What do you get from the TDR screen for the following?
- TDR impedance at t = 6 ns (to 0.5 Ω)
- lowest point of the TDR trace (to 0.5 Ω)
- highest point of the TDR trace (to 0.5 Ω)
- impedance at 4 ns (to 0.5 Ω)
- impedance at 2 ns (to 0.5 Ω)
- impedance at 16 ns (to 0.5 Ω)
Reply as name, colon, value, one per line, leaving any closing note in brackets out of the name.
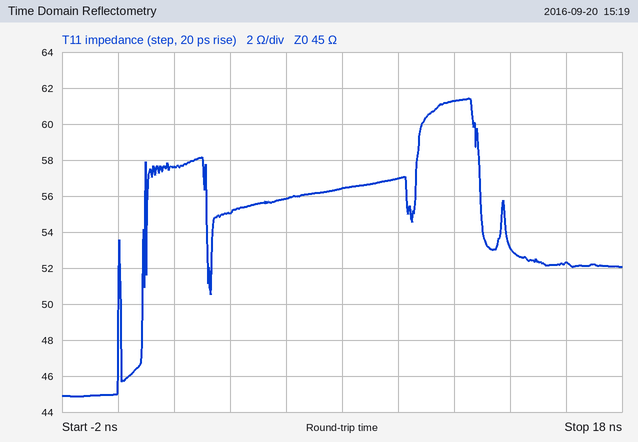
TDR impedance at t = 6 ns: 56.0 Ω
lowest point of the TDR trace: 45.0 Ω
highest point of the TDR trace: 61.5 Ω
impedance at 4 ns: 55.0 Ω
impedance at 2 ns: 57.5 Ω
impedance at 16 ns: 52.5 Ω
